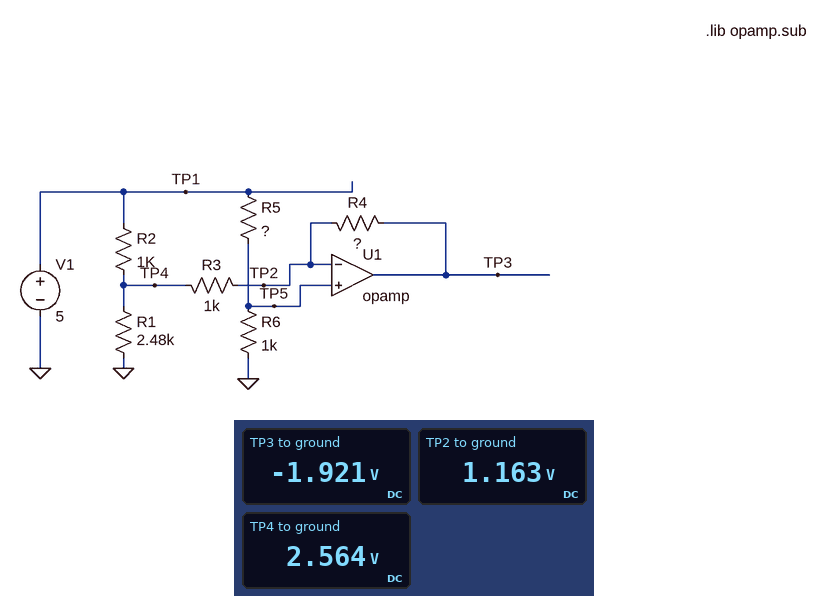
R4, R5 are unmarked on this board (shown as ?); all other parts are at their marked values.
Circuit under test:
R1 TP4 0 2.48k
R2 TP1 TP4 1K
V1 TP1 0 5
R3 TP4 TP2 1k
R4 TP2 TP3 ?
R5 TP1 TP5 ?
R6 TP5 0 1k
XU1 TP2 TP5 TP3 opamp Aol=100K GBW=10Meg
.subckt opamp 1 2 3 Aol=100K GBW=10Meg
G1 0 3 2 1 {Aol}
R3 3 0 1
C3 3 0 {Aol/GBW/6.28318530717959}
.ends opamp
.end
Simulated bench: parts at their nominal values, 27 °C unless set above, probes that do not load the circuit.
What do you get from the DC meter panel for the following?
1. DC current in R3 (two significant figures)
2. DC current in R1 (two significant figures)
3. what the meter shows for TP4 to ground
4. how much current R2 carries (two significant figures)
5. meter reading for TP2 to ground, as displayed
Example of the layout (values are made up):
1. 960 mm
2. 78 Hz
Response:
1. 1.4 mA
2. 1.0 mA
3. 2.564 V
4. 2.4 mA
5. 1.163 V
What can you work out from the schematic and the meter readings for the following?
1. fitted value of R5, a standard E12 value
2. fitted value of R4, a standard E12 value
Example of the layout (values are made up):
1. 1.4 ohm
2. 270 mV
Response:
1. 3.3 kΩ
2. 2.2 kΩ
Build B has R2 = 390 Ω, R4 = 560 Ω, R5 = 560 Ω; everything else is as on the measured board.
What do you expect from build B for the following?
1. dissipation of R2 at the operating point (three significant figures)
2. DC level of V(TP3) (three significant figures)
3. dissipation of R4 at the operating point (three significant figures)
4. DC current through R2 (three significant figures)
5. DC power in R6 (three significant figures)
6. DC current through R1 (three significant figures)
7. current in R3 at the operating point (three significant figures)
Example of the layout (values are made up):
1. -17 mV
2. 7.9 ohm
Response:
1. 2.37 mW
2. 2.74 V
3. 390 µW
4. 2.46 mA
5. 10.3 mW
6. 1.63 mA
7. 834 µA
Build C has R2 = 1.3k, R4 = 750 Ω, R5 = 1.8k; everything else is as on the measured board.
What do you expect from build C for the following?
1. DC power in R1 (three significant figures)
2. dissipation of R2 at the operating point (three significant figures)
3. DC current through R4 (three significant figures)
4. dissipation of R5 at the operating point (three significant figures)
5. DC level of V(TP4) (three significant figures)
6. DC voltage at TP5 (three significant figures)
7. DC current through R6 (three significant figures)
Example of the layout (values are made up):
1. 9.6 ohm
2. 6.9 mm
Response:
1. 2.71 mW
2. 4.46 mW
3. 807 µA
4. 5.74 mW
5. 2.59 V
6. 1.79 V
7. 1.79 mA
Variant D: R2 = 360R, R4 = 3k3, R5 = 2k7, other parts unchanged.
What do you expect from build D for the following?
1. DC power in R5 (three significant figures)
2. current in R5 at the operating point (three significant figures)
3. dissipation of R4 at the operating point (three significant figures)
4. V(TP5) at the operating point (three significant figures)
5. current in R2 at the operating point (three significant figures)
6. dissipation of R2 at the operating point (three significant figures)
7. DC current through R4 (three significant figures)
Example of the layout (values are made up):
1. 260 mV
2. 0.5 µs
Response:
1. 4.93 mW
2. 1.35 mA
3. 17.4 mW
4. 1.35 V
5. 3.76 mA
6. 5.10 mW
7. 2.29 mA
